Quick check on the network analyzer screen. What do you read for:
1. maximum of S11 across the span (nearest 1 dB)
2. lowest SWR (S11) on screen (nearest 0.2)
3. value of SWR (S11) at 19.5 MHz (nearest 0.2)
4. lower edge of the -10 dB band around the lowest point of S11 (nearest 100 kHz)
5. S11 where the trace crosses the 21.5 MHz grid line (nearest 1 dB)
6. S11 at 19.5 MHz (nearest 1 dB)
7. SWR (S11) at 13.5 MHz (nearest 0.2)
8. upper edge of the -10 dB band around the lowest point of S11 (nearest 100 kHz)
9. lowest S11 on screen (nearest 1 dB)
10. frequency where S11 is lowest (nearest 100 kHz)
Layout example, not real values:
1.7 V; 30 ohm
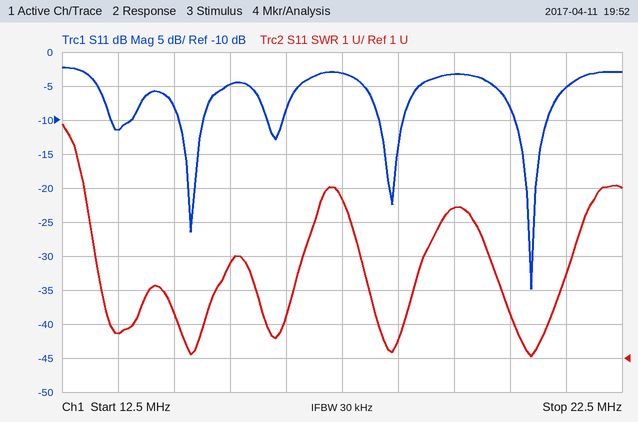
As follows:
-2 dB; 1.0; 5.4; 20.6 MHz; -5 dB; -3 dB; 1.8; 21.2 MHz; -35 dB; 20.9 MHz
